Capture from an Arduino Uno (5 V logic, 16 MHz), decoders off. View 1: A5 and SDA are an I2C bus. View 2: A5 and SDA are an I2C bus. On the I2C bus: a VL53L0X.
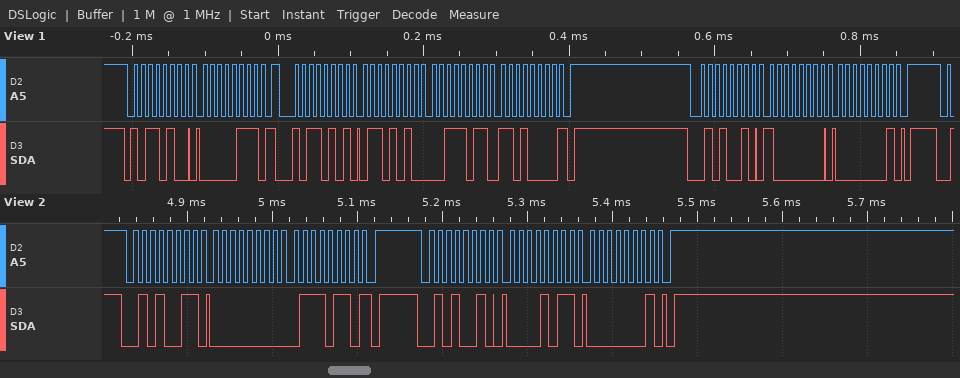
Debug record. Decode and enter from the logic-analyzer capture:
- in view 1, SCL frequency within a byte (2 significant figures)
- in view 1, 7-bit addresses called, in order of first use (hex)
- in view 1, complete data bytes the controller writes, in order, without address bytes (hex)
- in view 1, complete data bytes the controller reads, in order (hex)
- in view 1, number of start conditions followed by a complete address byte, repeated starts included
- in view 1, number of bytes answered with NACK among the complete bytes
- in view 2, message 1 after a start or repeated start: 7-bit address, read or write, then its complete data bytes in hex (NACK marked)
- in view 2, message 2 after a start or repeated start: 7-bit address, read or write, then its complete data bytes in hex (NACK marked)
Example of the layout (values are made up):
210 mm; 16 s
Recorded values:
100 kHz; 0x5A 0x29; 07 80 01; 6A 3B D0; 3; 1; 0x29 read: 00 76 NACK; 0x29 write: 0B 01
